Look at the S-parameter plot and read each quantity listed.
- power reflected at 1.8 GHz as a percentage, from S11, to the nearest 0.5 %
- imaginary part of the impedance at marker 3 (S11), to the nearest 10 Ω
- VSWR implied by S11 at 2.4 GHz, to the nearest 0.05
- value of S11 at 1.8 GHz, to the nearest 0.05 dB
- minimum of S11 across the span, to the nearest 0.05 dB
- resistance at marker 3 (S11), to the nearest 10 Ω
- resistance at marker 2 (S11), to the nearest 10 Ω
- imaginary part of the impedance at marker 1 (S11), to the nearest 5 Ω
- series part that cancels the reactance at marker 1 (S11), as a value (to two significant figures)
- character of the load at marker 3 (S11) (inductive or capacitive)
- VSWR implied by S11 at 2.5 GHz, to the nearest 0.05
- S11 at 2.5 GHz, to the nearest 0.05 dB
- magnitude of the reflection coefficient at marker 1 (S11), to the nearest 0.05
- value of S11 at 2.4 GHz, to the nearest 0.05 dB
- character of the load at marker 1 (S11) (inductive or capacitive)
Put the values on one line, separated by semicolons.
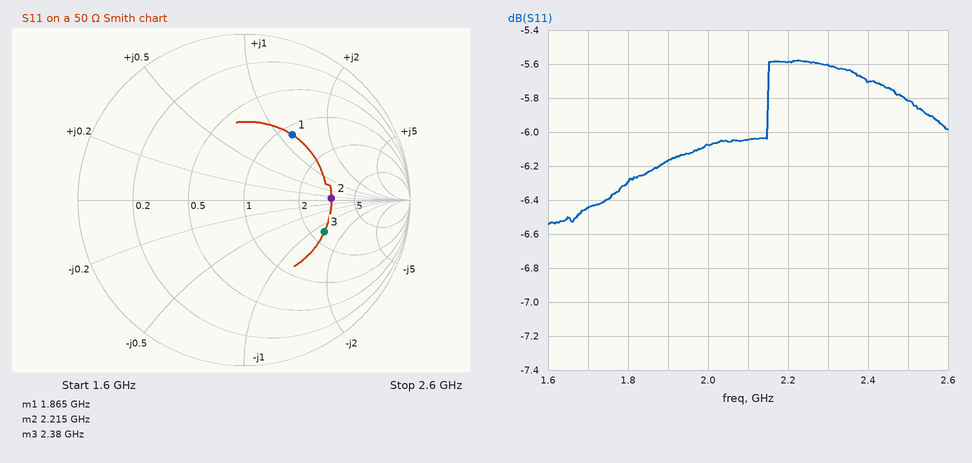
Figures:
23.5 %; -60 Ω; 3.15; -6.30 dB; -6.55 dB; 120 Ω; 160 Ω; +60 Ω; 1.4 pF; capacitive; 3.10; -5.80 dB; 0.50; -5.70 dB; inductive
